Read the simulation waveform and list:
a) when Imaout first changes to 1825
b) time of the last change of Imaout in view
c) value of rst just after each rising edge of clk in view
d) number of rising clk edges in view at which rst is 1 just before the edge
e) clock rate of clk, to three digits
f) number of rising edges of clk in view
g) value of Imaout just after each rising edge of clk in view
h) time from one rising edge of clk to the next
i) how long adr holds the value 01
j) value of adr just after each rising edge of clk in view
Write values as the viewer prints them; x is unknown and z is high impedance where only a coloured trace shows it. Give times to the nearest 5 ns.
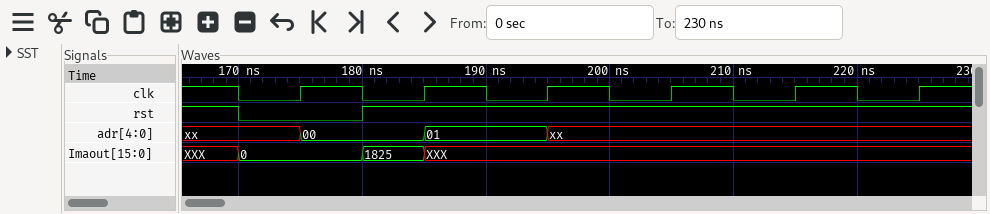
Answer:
180 ns
185 ns
0 1 1 1 1 1
5
100 MHz
6
0, XXX, XXX, XXX, XXX, XXX
10 ns
10 ns
00, 01, xx, xx, xx, xx
